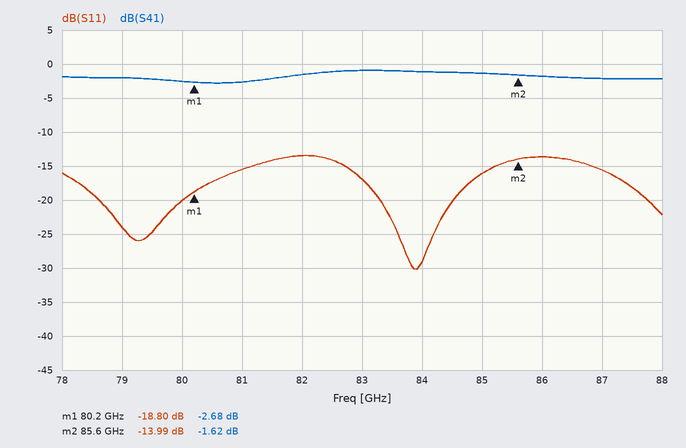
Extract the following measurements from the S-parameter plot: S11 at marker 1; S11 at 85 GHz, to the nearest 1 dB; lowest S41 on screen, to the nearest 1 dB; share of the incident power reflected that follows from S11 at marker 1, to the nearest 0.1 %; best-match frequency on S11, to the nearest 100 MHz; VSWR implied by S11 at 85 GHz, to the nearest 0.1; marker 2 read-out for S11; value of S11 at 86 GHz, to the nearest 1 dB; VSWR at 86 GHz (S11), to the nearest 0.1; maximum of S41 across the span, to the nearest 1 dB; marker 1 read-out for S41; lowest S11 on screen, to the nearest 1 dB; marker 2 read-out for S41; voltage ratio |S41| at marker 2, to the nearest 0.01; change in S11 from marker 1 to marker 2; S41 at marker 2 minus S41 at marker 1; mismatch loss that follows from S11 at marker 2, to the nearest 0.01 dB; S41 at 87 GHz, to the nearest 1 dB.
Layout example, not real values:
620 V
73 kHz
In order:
-18.80 dB
-16 dB
-3 dB
1.3 %
83.9 GHz
1.4
-13.99 dB
-14 dB
1.5
-1 dB
-2.68 dB
-30 dB
-1.62 dB
0.83
4.81 dB
1.06 dB
0.18 dB
-2 dB
